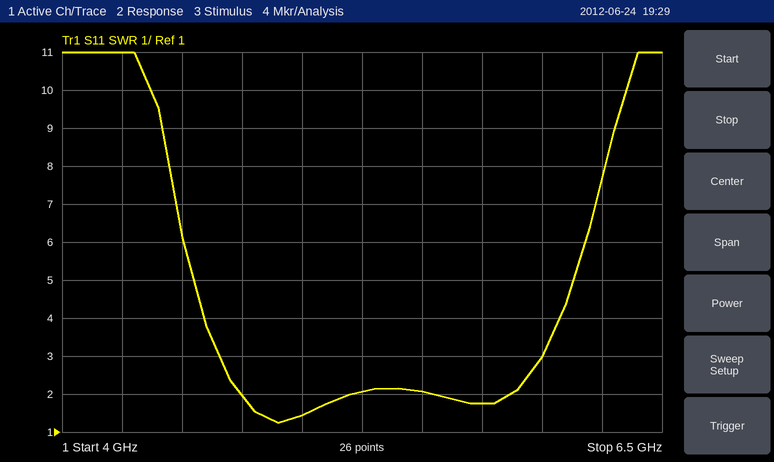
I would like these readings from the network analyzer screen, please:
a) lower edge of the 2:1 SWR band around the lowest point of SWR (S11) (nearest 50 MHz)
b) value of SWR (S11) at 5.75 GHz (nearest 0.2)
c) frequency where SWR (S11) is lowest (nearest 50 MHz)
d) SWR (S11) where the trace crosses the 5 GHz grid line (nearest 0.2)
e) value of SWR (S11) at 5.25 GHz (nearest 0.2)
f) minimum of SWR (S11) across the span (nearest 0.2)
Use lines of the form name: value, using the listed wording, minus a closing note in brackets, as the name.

lower edge of the 2:1 SWR band around the lowest point of SWR (S11): 4.75 GHz
value of SWR (S11) at 5.75 GHz: 1.8
frequency where SWR (S11) is lowest: 4.90 GHz
SWR (S11) where the trace crosses the 5 GHz grid line: 1.4
value of SWR (S11) at 5.25 GHz: 2.0
minimum of SWR (S11) across the span: 1.2
